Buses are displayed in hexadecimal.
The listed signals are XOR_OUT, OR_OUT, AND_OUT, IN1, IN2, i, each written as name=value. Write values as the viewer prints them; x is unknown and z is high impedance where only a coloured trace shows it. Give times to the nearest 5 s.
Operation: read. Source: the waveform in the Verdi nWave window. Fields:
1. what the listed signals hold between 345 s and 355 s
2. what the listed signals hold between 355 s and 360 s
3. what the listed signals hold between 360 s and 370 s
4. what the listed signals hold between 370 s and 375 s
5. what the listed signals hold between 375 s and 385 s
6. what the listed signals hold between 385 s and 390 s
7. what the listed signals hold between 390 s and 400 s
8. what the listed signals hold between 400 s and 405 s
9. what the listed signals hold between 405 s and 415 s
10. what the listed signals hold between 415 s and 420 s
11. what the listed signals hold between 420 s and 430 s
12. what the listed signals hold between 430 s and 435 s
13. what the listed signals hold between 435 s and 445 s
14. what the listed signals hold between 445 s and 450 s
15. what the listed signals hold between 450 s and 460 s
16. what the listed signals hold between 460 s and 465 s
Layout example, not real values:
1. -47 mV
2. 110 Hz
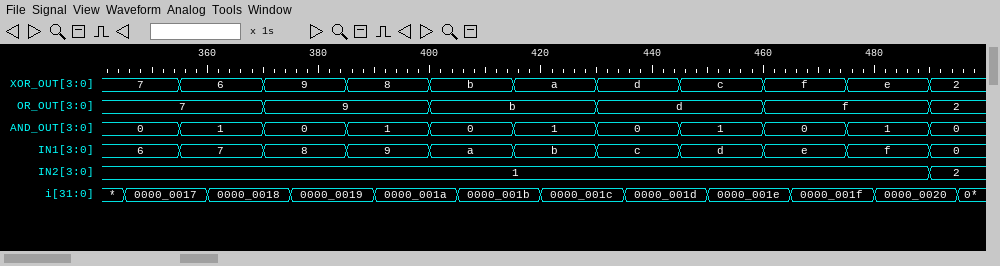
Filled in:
1. XOR_OUT=7, OR_OUT=7, AND_OUT=0, IN1=6, IN2=1, i=0000_0017
2. XOR_OUT=6, OR_OUT=7, AND_OUT=1, IN1=7, IN2=1, i=0000_0017
3. XOR_OUT=6, OR_OUT=7, AND_OUT=1, IN1=7, IN2=1, i=0000_0018
4. XOR_OUT=9, OR_OUT=9, AND_OUT=0, IN1=8, IN2=1, i=0000_0018
5. XOR_OUT=9, OR_OUT=9, AND_OUT=0, IN1=8, IN2=1, i=0000_0019
6. XOR_OUT=8, OR_OUT=9, AND_OUT=1, IN1=9, IN2=1, i=0000_0019
7. XOR_OUT=8, OR_OUT=9, AND_OUT=1, IN1=9, IN2=1, i=0000_001a
8. XOR_OUT=b, OR_OUT=b, AND_OUT=0, IN1=a, IN2=1, i=0000_001a
9. XOR_OUT=b, OR_OUT=b, AND_OUT=0, IN1=a, IN2=1, i=0000_001b
10. XOR_OUT=a, OR_OUT=b, AND_OUT=1, IN1=b, IN2=1, i=0000_001b
11. XOR_OUT=a, OR_OUT=b, AND_OUT=1, IN1=b, IN2=1, i=0000_001c
12. XOR_OUT=d, OR_OUT=d, AND_OUT=0, IN1=c, IN2=1, i=0000_001c
13. XOR_OUT=d, OR_OUT=d, AND_OUT=0, IN1=c, IN2=1, i=0000_001d
14. XOR_OUT=c, OR_OUT=d, AND_OUT=1, IN1=d, IN2=1, i=0000_001d
15. XOR_OUT=c, OR_OUT=d, AND_OUT=1, IN1=d, IN2=1, i=0000_001e
16. XOR_OUT=f, OR_OUT=f, AND_OUT=0, IN1=e, IN2=1, i=0000_001e
